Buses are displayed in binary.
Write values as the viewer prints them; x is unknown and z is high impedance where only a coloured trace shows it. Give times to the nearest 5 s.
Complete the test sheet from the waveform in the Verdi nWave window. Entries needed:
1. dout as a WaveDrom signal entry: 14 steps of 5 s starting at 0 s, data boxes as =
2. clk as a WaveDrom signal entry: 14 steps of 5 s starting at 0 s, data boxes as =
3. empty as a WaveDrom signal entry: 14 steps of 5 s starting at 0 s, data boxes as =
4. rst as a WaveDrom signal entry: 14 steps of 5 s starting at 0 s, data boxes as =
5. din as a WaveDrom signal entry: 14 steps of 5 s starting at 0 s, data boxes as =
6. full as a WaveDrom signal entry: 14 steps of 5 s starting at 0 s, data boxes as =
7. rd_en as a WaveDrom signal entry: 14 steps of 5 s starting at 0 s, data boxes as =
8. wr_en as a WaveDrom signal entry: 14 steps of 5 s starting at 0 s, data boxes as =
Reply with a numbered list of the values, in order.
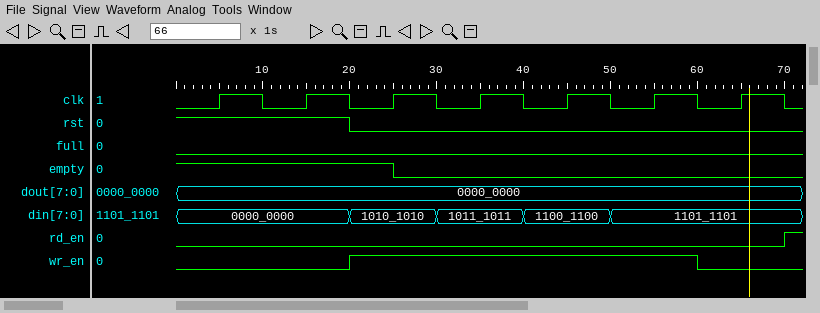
1. {name: 'dout', wave: '=.............', data: '0000_0000'}
2. {name: 'clk', wave: '01010101010101'}
3. {name: 'empty', wave: '1....0........'}
4. {name: 'rst', wave: '1...0.........'}
5. {name: 'din', wave: '=...=.=.=.=...', data: '0000_0000 1010_1010 1011_1011 1100_1100 1101_1101'}
6. {name: 'full', wave: '0.............'}
7. {name: 'rd_en', wave: '0.............'}
8. {name: 'wr_en', wave: '0...1.......0.'}
